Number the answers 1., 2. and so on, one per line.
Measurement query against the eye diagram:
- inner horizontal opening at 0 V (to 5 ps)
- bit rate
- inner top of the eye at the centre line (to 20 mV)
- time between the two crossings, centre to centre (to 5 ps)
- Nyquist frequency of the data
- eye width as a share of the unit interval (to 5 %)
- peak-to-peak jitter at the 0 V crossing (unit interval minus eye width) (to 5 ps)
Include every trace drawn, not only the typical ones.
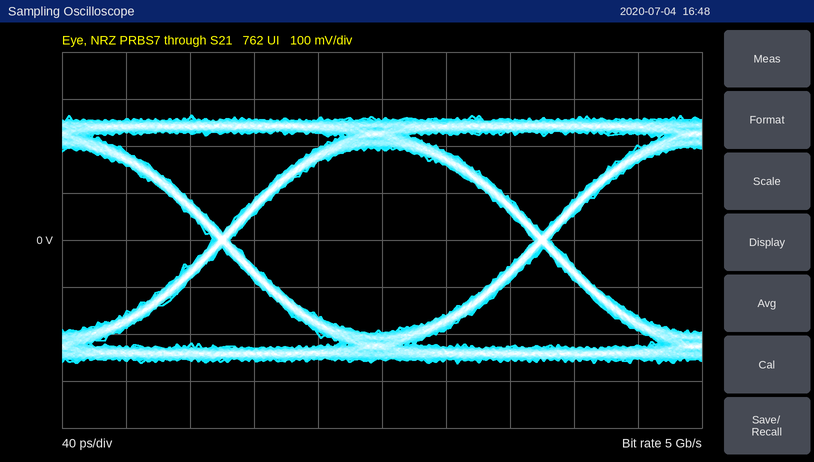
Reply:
1. 190 ps
2. 5 Gb/s
3. 200 mV
4. 200 ps
5. 2.5 GHz
6. 95 %
7. 10 ps
